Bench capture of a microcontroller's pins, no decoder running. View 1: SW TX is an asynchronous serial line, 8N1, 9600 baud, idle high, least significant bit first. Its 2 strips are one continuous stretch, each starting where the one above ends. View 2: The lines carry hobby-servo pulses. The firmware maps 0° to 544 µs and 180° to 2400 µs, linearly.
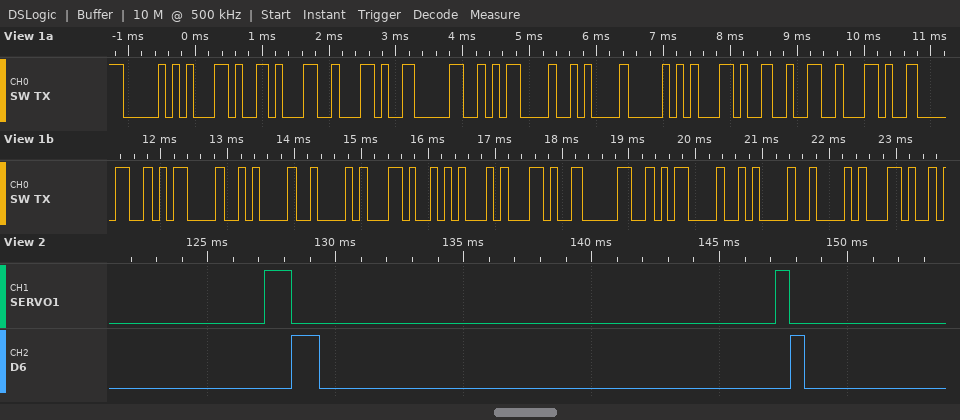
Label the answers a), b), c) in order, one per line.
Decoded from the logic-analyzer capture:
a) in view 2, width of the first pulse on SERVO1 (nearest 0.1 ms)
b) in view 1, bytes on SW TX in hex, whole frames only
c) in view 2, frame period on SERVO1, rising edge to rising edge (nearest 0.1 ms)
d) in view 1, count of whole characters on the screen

a) 1.1 ms
b) 50 2C 31 2C 30 0D 0A 50 2C 32 2C 30 0D 0A 42 2C 45 2C 30 0D 0A 42 2C
c) 20.0 ms
d) 23
